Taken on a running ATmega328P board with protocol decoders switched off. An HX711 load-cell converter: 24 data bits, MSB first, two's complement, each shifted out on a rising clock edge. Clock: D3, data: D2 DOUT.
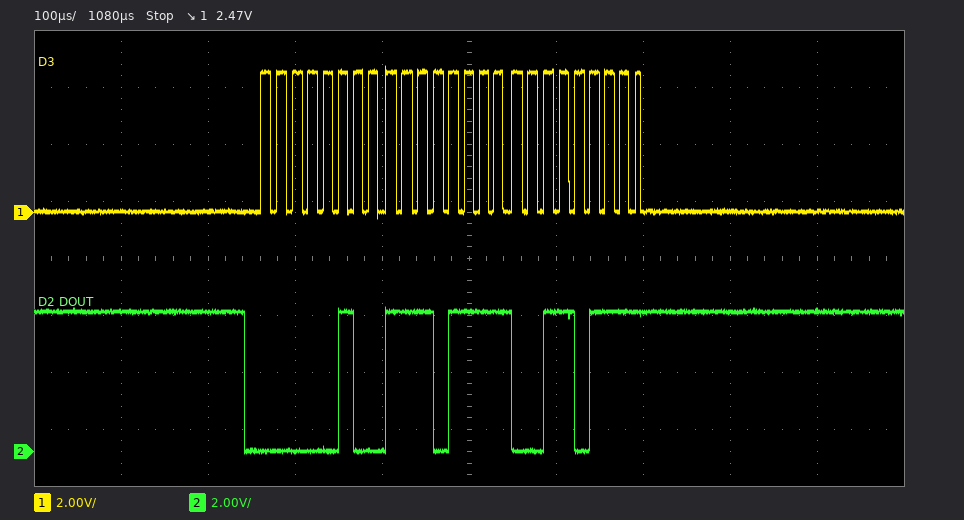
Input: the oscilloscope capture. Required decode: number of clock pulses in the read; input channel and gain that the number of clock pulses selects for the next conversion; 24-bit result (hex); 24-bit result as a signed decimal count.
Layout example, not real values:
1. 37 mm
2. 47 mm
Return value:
1. 25
2. channel A, gain 128
3. 0x04EF37
4. 323383
